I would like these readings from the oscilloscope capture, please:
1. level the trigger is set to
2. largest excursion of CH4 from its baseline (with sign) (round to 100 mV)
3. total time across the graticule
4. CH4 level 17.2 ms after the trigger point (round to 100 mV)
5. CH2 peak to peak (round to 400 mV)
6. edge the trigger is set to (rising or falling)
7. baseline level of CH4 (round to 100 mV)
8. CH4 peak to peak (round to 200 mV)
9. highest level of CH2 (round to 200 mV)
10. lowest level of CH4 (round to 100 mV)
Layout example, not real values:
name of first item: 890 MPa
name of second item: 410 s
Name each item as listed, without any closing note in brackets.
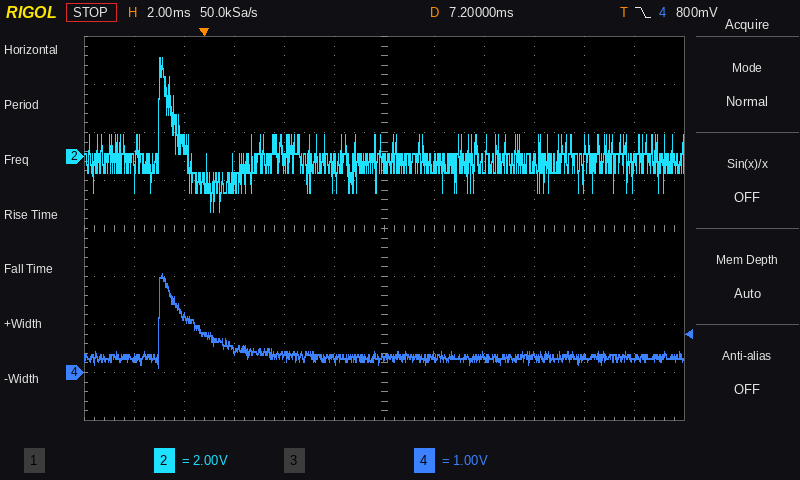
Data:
level the trigger is set to: 800 mV
largest excursion of CH4 from its baseline (with sign): +1.7 V
total time across the graticule: 24 ms
CH4 level 17.2 ms after the trigger point: 300 mV
CH2 peak to peak: 6.4 V
edge the trigger is set to: falling
baseline level of CH4: 300 mV
CH4 peak to peak: 2.0 V
highest level of CH2: 4.2 V
lowest level of CH4: 100 mV
